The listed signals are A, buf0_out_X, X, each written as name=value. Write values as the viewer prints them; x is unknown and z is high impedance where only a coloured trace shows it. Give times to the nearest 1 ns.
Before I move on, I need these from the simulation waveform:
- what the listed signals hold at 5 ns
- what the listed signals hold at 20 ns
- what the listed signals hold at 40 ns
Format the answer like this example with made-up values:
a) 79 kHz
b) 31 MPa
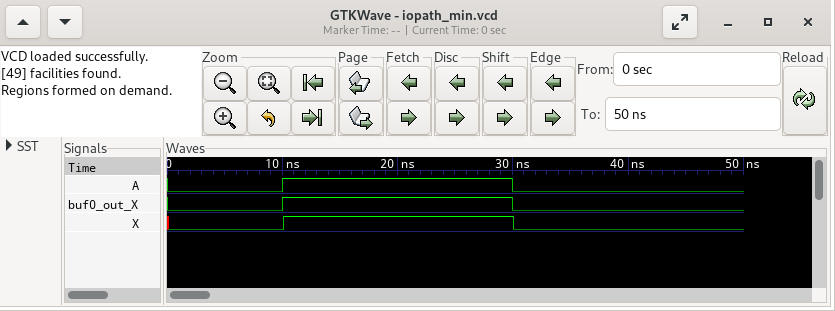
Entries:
a) A=0, buf0_out_X=0, X=0
b) A=1, buf0_out_X=1, X=1
c) A=0, buf0_out_X=0, X=0
